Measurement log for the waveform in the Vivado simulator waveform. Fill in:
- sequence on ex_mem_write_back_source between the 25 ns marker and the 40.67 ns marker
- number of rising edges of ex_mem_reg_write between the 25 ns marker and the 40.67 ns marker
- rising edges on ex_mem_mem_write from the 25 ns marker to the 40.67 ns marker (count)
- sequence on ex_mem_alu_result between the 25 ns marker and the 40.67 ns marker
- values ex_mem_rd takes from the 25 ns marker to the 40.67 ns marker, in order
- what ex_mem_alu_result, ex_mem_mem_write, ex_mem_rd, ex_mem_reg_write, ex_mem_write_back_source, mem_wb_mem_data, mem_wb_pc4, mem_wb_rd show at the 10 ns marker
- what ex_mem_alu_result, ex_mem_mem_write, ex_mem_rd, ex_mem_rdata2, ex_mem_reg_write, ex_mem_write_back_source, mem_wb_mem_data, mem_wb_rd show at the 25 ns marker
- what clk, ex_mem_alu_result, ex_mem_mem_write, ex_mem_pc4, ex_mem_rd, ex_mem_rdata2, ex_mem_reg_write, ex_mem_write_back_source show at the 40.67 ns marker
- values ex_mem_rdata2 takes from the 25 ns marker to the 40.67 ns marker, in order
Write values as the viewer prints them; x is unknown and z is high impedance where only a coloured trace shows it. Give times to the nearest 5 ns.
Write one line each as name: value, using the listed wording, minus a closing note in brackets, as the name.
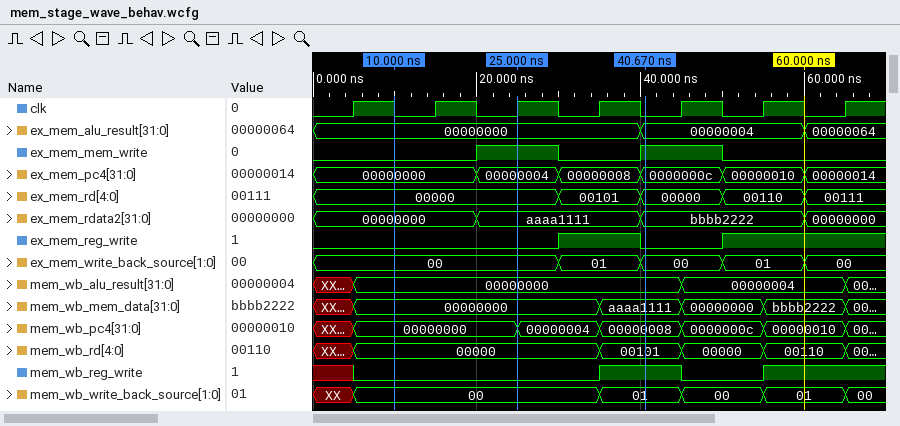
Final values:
sequence on ex_mem_write_back_source between the 25 ns marker and the 40.67 ns marker: 00, 01, 00
number of rising edges of ex_mem_reg_write between the 25 ns marker and the 40.67 ns marker: 1
rising edges on ex_mem_mem_write from the 25 ns marker to the 40.67 ns marker: 1
sequence on ex_mem_alu_result between the 25 ns marker and the 40.67 ns marker: 00000000, 00000004
values ex_mem_rd takes from the 25 ns marker to the 40.67 ns marker, in order: 00000, 00101, 00000
what ex_mem_alu_result, ex_mem_mem_write, ex_mem_rd, ex_mem_reg_write, ex_mem_write_back_source, mem_wb_mem_data, mem_wb_pc4, mem_wb_rd show at the 10 ns marker: ex_mem_alu_result=00000000, ex_mem_mem_write=0, ex_mem_rd=00000, ex_mem_reg_write=0, ex_mem_write_back_source=00, mem_wb_mem_data=00000000, mem_wb_pc4=00000000, mem_wb_rd=00000
what ex_mem_alu_result, ex_mem_mem_write, ex_mem_rd, ex_mem_rdata2, ex_mem_reg_write, ex_mem_write_back_source, mem_wb_mem_data, mem_wb_rd show at the 25 ns marker: ex_mem_alu_result=00000000, ex_mem_mem_write=1, ex_mem_rd=00000, ex_mem_rdata2=aaaa1111, ex_mem_reg_write=0, ex_mem_write_back_source=00, mem_wb_mem_data=00000000, mem_wb_rd=00000
what clk, ex_mem_alu_result, ex_mem_mem_write, ex_mem_pc4, ex_mem_rd, ex_mem_rdata2, ex_mem_reg_write, ex_mem_write_back_source show at the 40.67 ns marker: clk=0, ex_mem_alu_result=00000004, ex_mem_mem_write=1, ex_mem_pc4=0000000c, ex_mem_rd=00000, ex_mem_rdata2=bbbb2222, ex_mem_reg_write=0, ex_mem_write_back_source=00
values ex_mem_rdata2 takes from the 25 ns marker to the 40.67 ns marker, in order: aaaa1111, bbbb2222
